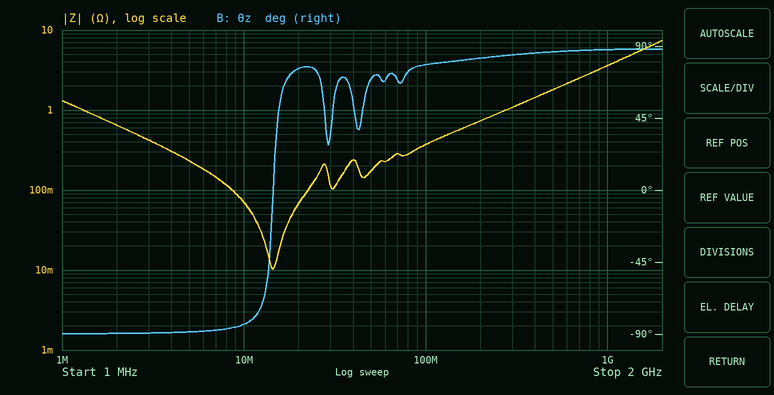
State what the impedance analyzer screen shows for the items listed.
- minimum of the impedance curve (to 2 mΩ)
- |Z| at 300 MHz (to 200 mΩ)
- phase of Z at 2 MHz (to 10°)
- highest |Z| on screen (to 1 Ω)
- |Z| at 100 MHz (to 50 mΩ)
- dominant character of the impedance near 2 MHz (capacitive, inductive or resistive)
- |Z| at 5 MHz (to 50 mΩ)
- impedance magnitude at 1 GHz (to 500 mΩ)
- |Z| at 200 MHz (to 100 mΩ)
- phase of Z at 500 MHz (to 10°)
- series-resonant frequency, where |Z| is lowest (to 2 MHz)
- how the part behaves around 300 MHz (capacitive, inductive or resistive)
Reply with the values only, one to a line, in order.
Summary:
10 mΩ
1.0 Ω
-90°
7 Ω
350 mΩ
capacitive
250 mΩ
3.5 Ω
700 mΩ
90°
14 MHz
inductive
